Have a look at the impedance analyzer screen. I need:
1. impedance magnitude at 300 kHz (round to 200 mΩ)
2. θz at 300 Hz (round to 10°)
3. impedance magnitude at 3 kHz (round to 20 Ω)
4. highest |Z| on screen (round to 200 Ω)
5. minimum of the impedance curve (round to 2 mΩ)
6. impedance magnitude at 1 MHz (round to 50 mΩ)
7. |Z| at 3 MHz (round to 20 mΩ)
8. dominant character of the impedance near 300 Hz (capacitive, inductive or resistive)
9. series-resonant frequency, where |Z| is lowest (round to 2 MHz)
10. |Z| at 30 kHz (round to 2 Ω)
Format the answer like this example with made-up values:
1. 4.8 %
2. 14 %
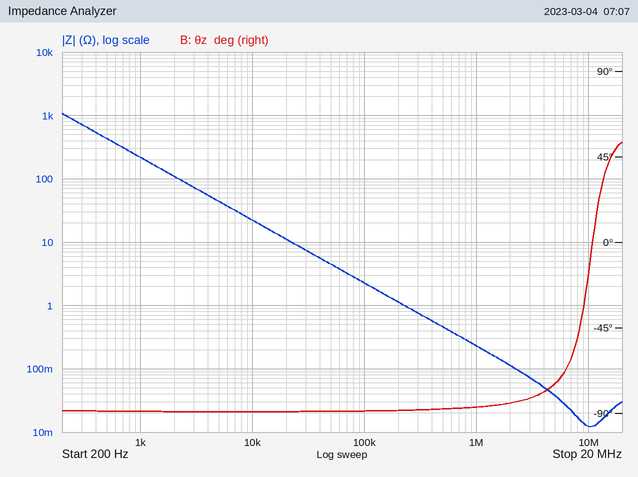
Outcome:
1. 800 mΩ
2. -90°
3. 80 Ω
4. 1.0 kΩ
5. 12 mΩ
6. 250 mΩ
7. 80 mΩ
8. capacitive
9. 10 MHz
10. 8 Ω
